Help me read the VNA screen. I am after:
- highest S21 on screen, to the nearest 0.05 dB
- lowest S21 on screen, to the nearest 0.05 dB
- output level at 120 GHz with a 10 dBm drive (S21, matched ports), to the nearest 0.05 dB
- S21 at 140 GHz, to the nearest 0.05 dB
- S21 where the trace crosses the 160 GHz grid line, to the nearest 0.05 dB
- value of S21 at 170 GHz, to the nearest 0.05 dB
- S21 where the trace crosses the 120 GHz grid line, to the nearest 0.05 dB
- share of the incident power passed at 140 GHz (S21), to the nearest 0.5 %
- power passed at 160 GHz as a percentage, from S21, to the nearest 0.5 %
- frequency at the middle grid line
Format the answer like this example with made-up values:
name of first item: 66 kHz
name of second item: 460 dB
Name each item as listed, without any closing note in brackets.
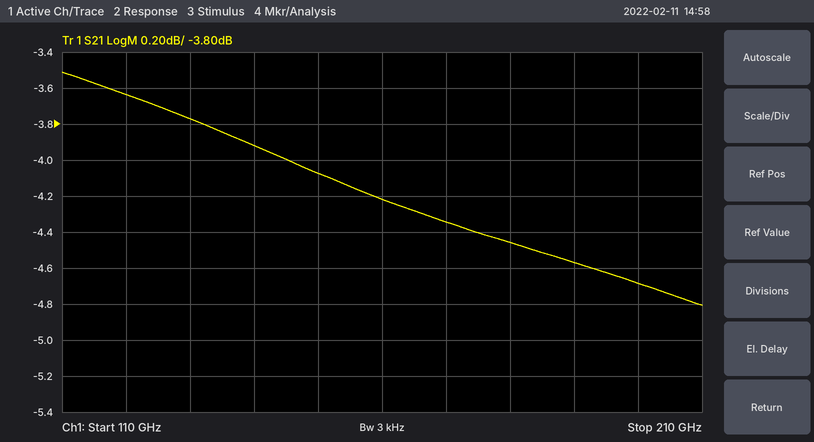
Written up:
highest S21 on screen, to the nearest 0.05 dB: -3.50 dB
lowest S21 on screen, to the nearest 0.05 dB: -4.80 dB
output level at 120 GHz with a 10 dBm drive (S21, matched ports), to the nearest 0.05 dB: 6.35 dBm
S21 at 140 GHz, to the nearest 0.05 dB: -3.90 dB
S21 where the trace crosses the 160 GHz grid line, to the nearest 0.05 dB: -4.20 dB
value of S21 at 170 GHz, to the nearest 0.05 dB: -4.35 dB
S21 where the trace crosses the 120 GHz grid line, to the nearest 0.05 dB: -3.65 dB
share of the incident power passed at 140 GHz (S21), to the nearest 0.5 %: 40.5 %
power passed at 160 GHz as a percentage, from S21, to the nearest 0.5 %: 38.0 %
frequency at the middle grid line: 160 GHz
